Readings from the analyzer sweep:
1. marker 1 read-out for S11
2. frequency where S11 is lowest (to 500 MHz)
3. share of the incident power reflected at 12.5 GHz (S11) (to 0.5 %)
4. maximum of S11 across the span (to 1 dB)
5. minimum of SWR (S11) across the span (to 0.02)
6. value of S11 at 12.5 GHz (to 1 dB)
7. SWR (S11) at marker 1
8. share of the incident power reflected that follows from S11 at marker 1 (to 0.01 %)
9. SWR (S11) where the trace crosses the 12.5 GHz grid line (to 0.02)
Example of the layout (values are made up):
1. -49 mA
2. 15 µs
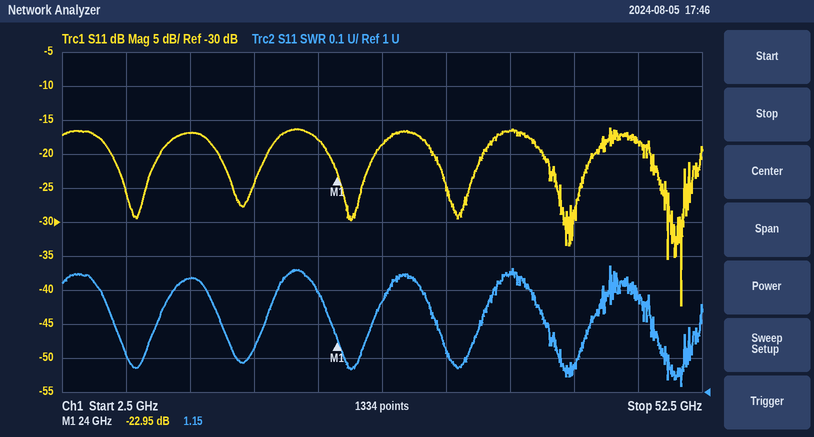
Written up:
1. -22.95 dB
2. 51.0 GHz
3. 2.0 %
4. -16 dB
5. 1.02
6. -17 dB
7. 1.15
8. 0.51 %
9. 1.34
